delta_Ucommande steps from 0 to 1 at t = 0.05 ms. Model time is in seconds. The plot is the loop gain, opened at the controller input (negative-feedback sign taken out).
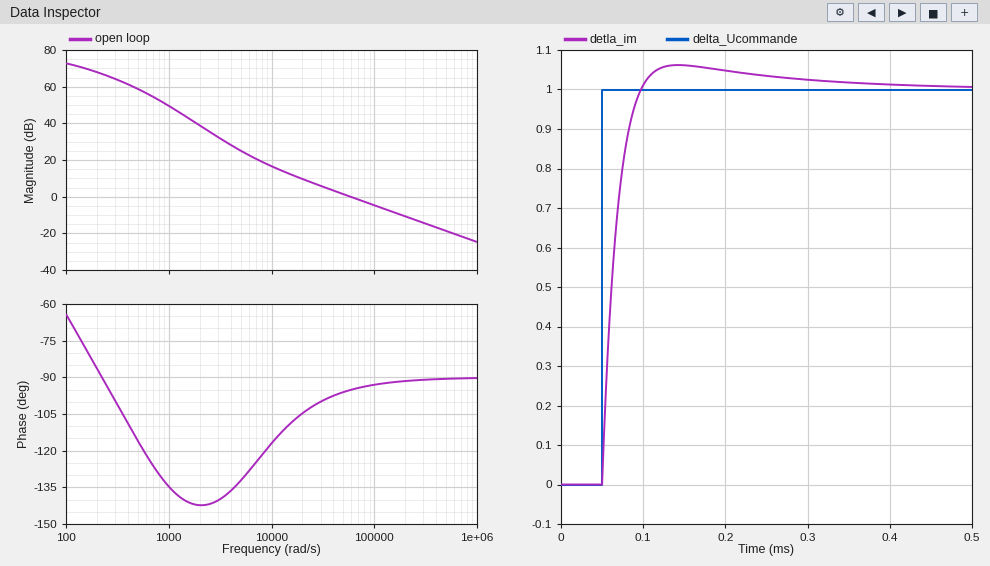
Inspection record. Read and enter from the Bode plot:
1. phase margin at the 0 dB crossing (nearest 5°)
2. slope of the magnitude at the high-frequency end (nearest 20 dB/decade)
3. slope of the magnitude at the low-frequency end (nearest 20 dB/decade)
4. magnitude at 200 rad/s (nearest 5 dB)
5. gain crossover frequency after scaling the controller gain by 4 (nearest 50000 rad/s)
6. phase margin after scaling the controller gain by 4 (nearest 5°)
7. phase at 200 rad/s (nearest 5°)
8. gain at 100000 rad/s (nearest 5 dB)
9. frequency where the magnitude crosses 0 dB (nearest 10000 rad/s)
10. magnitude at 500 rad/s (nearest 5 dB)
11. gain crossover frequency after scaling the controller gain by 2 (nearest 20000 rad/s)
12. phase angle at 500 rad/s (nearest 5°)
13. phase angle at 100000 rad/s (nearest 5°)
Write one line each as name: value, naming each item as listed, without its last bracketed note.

phase margin at the 0 dB crossing: 85°
slope of the magnitude at the high-frequency end: -20 dB/decade
slope of the magnitude at the low-frequency end: -20 dB/decade
magnitude at 200 rad/s: 70 dB
gain crossover frequency after scaling the controller gain by 4: 250000 rad/s
phase margin after scaling the controller gain by 4: 90°
phase at 200 rad/s: -85°
gain at 100000 rad/s: -5 dB
frequency where the magnitude crosses 0 dB: 60000 rad/s
magnitude at 500 rad/s: 60 dB
gain crossover frequency after scaling the controller gain by 2: 120000 rad/s
phase angle at 500 rad/s: -115°
phase angle at 100000 rad/s: -95°
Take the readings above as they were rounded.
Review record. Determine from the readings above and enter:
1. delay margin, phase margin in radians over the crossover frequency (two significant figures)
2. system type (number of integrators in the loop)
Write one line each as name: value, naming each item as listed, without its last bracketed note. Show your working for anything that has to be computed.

delay margin, phase margin in radians over the crossover frequency: 85 × π / 180 / 60000 = 0.000025 s
system type: 1
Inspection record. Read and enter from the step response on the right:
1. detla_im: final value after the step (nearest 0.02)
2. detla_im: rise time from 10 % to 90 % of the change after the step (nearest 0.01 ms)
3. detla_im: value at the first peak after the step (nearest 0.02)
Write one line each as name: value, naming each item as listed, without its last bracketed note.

detla_im: final value after the step: 1.00
detla_im: rise time from 10 % to 90 % of the change after the step: 0.03 ms
detla_im: value at the first peak after the step: 1.06
